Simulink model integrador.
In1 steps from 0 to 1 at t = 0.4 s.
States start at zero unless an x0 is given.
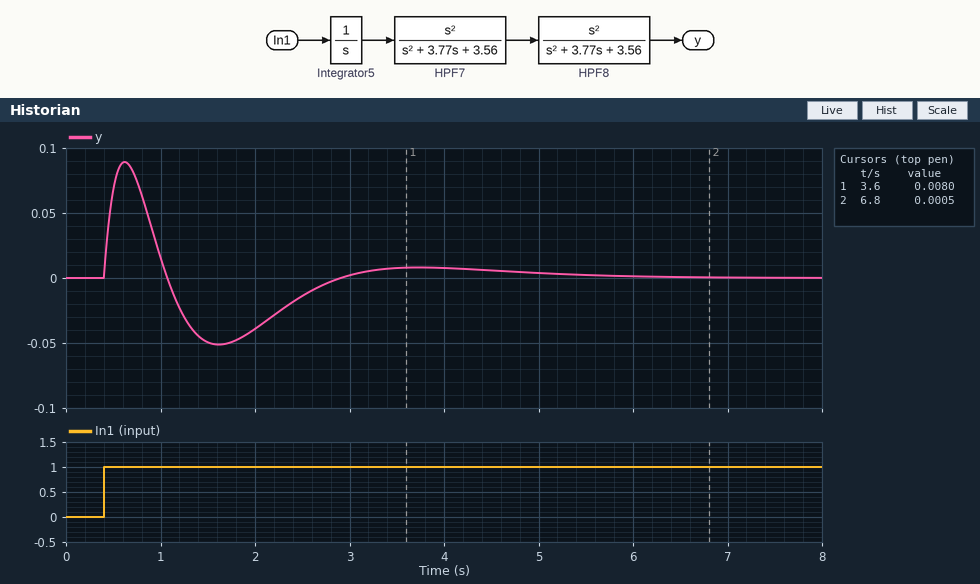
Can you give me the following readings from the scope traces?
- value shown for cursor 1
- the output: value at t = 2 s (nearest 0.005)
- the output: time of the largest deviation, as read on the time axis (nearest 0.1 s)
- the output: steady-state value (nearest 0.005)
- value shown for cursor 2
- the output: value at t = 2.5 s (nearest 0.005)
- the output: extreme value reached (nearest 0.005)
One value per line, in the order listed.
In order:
0.0080
-0.040
0.6 s
0.000
0.0005
-0.015
0.090
